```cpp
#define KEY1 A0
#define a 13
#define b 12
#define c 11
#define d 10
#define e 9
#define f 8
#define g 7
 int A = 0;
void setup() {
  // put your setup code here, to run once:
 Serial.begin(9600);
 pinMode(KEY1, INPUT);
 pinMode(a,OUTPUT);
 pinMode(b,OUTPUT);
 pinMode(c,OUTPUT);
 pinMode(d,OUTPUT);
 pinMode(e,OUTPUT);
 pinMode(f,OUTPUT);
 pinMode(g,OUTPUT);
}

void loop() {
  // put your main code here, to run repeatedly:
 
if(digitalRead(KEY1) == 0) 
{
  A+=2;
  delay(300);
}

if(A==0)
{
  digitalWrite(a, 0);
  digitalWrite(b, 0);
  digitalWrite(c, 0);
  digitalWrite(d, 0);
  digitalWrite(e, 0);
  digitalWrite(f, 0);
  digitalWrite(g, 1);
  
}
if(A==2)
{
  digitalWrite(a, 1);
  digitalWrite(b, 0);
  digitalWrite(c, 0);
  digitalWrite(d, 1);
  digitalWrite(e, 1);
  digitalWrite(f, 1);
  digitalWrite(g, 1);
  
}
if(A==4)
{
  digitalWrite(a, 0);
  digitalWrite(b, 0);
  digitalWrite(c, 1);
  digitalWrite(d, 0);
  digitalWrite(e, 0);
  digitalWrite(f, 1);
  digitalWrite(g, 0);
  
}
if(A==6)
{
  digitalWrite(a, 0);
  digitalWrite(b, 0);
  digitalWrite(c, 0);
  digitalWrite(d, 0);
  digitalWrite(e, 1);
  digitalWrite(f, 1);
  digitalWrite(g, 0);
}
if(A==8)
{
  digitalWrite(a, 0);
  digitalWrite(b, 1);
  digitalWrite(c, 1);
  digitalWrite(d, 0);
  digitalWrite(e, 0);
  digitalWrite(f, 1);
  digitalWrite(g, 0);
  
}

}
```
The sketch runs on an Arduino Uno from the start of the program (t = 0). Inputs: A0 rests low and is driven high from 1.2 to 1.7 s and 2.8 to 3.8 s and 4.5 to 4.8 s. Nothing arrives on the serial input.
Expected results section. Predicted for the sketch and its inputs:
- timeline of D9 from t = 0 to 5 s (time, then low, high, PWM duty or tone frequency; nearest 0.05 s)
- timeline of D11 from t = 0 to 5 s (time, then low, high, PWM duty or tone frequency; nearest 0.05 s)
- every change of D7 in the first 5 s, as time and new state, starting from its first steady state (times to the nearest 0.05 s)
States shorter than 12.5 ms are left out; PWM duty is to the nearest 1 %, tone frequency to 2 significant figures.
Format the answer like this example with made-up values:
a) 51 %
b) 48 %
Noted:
a) 0 s low; 0.3 s high; 0.6 s low; 0.9 s high; 1.2 s low
b) 0 s low; 0.6 s high; 0.9 s low; 1.2 s high
c) 0 s low; 0.3 s high; 0.6 s low
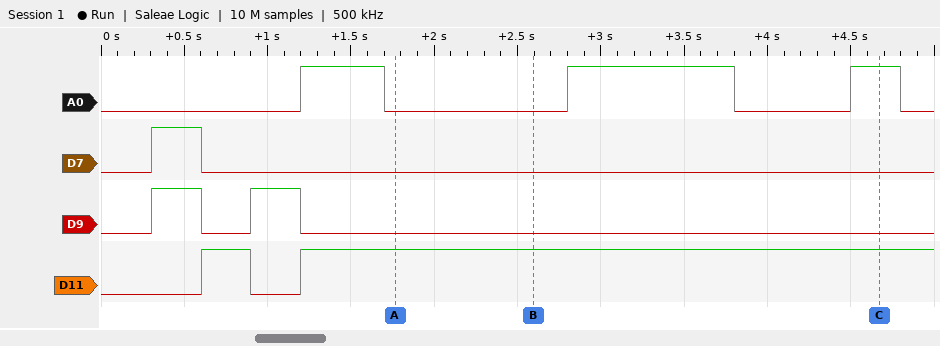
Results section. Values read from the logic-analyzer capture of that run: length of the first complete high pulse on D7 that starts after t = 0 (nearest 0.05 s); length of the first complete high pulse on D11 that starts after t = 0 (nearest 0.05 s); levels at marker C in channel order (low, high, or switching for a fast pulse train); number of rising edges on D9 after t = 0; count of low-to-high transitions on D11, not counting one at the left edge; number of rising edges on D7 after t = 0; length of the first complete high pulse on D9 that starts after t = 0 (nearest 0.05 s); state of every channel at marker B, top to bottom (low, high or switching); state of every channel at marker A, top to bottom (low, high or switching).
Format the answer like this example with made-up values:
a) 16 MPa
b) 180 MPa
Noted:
a) 0.30 s
b) 0.30 s
c) A0 high, D7 low, D9 low, D11 high
d) 2
e) 2
f) 1
g) 0.30 s
h) A0 low, D7 low, D9 low, D11 high
i) A0 low, D7 low, D9 low, D11 high
